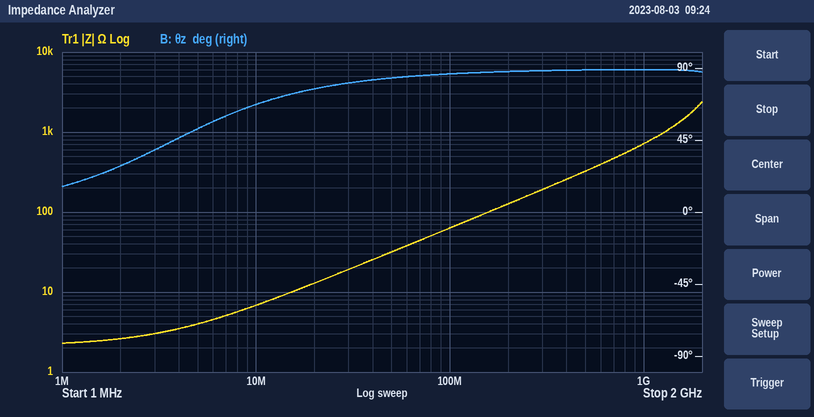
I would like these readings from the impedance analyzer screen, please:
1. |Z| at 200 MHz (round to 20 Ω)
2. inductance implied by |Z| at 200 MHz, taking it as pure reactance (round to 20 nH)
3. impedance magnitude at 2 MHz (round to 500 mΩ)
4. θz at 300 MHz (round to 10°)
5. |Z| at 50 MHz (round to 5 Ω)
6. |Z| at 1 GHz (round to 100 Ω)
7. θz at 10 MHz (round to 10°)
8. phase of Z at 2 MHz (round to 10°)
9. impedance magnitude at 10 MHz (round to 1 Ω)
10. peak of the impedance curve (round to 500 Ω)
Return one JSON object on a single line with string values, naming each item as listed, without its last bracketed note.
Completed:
{"|Z| at 200 MHz": "120 Ω", "inductance implied by |Z| at 200 MHz, taking it as pure reactance": "100 nH", "impedance magnitude at 2 MHz": "2.5 Ω", "θz at 300 MHz": "90°", "|Z| at 50 MHz": "30 Ω", "|Z| at 1 GHz": "700 Ω", "θz at 10 MHz": "70°", "phase of Z at 2 MHz": "30°", "impedance magnitude at 10 MHz": "7 Ω", "peak of the impedance curve": "2.5 kΩ"}
